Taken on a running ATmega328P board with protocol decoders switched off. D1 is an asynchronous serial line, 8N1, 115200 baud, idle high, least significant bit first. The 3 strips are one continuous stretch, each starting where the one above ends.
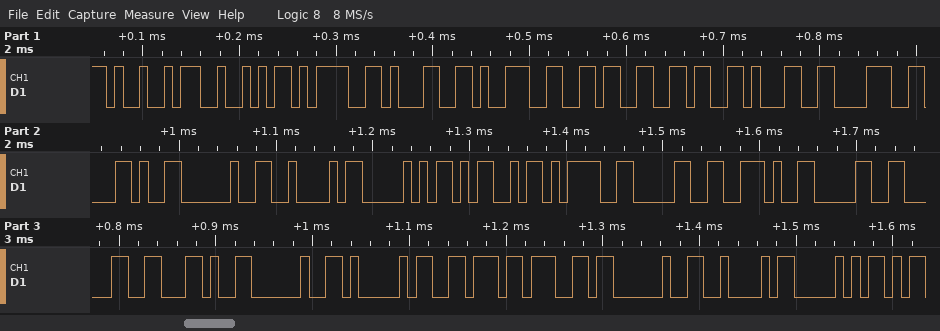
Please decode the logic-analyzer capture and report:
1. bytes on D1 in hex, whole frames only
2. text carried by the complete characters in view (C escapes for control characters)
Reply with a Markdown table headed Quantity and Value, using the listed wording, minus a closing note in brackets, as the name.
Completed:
| Quantity | Value |
|---|---|
| bytes on D1 in hex, whole frames only | 49 52 3D 31 39 36 36 31 38 2C 20 42 50 4D 3D 30 2E 30 30 2C 20 41 76 67 20 42 50 |
| text carried by the complete characters in view | "IR=196618, BPM=0.00, Avg BP" |
